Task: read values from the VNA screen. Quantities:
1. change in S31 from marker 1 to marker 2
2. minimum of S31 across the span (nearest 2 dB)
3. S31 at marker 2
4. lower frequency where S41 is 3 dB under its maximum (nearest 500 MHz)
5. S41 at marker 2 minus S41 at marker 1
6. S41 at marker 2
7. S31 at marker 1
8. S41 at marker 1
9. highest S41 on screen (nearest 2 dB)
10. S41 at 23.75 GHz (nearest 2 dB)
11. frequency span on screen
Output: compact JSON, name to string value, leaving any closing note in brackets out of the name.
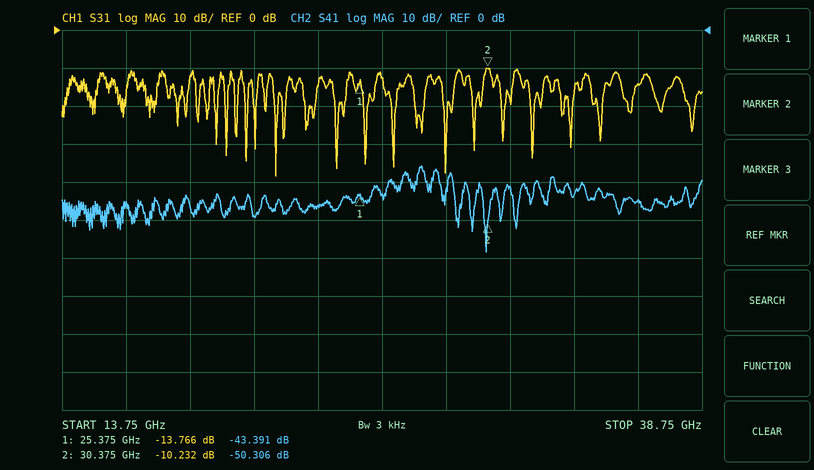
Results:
{"change in S31 from marker 1 to marker 2": "3.534 dB", "minimum of S31 across the span": "-38 dB", "S31 at marker 2": "-10.232 dB", "lower frequency where S41 is 3 dB under its maximum": "27.5 GHz", "S41 at marker 2 minus S41 at marker 1": "-6.915 dB", "S41 at marker 2": "-50.306 dB", "S31 at marker 1": "-13.766 dB", "S41 at marker 1": "-43.391 dB", "highest S41 on screen": "-36 dB", "S41 at 23.75 GHz": "-46 dB", "frequency span on screen": "25 GHz"}
